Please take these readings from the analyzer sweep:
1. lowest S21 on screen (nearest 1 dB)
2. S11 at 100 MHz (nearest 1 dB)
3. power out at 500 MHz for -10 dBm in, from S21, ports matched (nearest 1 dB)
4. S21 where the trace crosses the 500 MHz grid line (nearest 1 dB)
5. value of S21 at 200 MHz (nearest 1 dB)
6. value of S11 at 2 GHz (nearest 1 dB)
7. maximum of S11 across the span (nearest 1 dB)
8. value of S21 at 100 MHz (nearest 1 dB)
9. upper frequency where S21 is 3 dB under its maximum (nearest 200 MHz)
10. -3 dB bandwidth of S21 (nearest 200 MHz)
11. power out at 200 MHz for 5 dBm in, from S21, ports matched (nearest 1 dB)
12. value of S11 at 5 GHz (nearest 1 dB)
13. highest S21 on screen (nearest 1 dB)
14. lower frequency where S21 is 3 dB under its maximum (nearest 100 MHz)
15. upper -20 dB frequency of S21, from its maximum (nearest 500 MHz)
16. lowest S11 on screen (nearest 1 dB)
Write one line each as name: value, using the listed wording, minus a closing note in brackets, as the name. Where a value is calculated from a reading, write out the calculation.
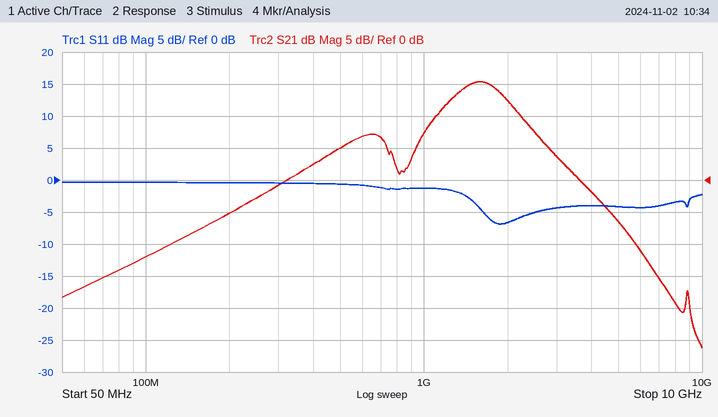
lowest S21 on screen: -26 dB
S11 at 100 MHz: 0 dB
power out at 500 MHz for -10 dBm in, from S21, ports matched: -10 dBm + (5 dB) = -5 dBm
S21 where the trace crosses the 500 MHz grid line: 5 dB
value of S21 at 200 MHz: -5 dB
value of S11 at 2 GHz: -7 dB
maximum of S11 across the span: 0 dB
value of S21 at 100 MHz: -12 dB
upper frequency where S21 is 3 dB under its maximum: 2.0 GHz
-3 dB bandwidth of S21: 2.0 GHz − 1.2 GHz = 800 MHz
power out at 200 MHz for 5 dBm in, from S21, ports matched: 5 dBm + (-5 dB) = 0 dBm
value of S11 at 5 GHz: -4 dB
highest S21 on screen: 15 dB
lower frequency where S21 is 3 dB under its maximum: 1.2 GHz
upper -20 dB frequency of S21, from its maximum: 4.5 GHz
lowest S11 on screen: -7 dB
